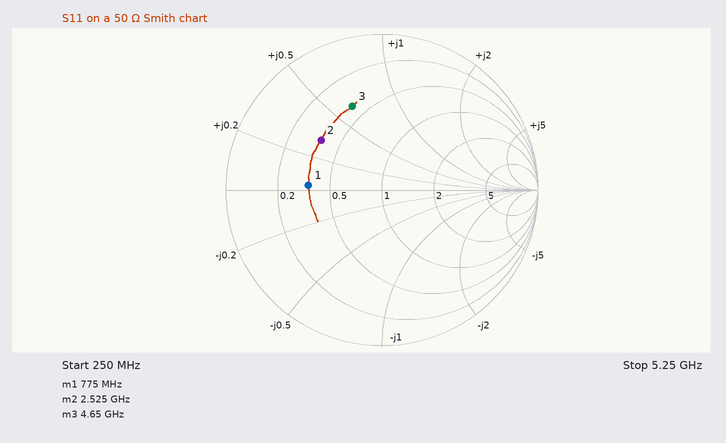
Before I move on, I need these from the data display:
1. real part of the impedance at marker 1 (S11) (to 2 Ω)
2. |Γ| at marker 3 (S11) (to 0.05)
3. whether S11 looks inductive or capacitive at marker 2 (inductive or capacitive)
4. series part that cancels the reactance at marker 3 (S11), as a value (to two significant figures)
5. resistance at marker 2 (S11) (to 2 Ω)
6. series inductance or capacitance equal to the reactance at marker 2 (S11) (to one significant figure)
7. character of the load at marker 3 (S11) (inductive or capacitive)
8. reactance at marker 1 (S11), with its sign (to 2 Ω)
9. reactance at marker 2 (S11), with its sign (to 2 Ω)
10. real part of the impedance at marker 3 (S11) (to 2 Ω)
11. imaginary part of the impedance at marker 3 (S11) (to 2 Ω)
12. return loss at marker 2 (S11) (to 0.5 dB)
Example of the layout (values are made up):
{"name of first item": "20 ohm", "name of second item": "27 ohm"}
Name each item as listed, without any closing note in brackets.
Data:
{"real part of the impedance at marker 1 (S11)": "18 Ω", "|Γ| at marker 3 (S11)": "0.55", "whether S11 looks inductive or capacitive at marker 2": "inductive", "series part that cancels the reactance at marker 3 (S11), as a value": "1.1 pF", "resistance at marker 2 (S11)": "18 Ω", "series inductance or capacitance equal to the reactance at marker 2 (S11)": "1.0 nH", "character of the load at marker 3 (S11)": "inductive", "reactance at marker 1 (S11), with its sign": "+2 Ω", "reactance at marker 2 (S11), with its sign": "+16 Ω", "real part of the impedance at marker 3 (S11)": "20 Ω", "imaginary part of the impedance at marker 3 (S11)": "+32 Ω", "return loss at marker 2 (S11)": "6.0 dB"}
